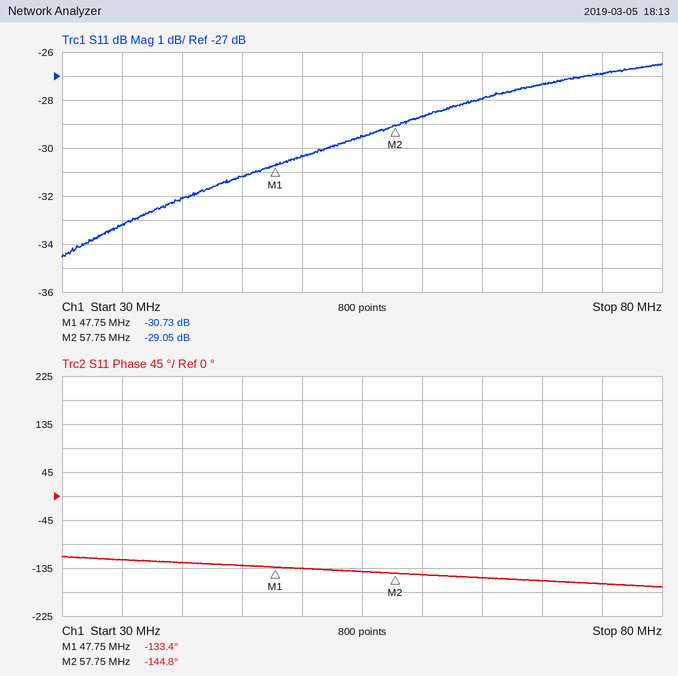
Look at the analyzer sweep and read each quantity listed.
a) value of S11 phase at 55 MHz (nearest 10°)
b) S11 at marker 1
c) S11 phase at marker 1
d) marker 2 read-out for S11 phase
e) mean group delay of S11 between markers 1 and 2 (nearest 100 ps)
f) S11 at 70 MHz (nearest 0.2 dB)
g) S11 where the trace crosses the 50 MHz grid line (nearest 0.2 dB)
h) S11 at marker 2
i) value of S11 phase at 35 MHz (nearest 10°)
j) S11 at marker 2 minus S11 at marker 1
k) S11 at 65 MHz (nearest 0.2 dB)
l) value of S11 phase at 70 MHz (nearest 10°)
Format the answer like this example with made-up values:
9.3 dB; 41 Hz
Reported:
-140°; -30.73 dB; -133.4°; -144.8°; 3.2 ns; -27.4 dB; -30.4 dB; -29.05 dB; -120°; 1.68 dB; -28.0 dB; -160°
